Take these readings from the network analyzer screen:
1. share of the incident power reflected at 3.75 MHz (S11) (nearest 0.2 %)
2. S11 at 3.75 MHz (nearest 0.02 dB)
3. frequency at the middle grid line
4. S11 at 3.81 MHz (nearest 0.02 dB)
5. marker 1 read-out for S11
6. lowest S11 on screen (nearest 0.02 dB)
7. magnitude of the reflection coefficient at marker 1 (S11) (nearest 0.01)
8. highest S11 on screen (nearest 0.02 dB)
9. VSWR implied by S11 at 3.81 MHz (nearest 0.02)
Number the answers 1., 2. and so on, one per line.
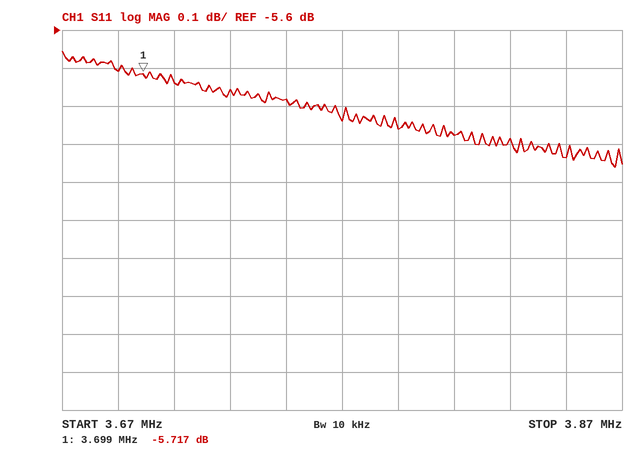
1. 26.4 %
2. -5.78 dB
3. 3.77 MHz
4. -5.88 dB
5. -5.717 dB
6. -5.96 dB
7. 0.52
8. -5.66 dB
9. 3.06
